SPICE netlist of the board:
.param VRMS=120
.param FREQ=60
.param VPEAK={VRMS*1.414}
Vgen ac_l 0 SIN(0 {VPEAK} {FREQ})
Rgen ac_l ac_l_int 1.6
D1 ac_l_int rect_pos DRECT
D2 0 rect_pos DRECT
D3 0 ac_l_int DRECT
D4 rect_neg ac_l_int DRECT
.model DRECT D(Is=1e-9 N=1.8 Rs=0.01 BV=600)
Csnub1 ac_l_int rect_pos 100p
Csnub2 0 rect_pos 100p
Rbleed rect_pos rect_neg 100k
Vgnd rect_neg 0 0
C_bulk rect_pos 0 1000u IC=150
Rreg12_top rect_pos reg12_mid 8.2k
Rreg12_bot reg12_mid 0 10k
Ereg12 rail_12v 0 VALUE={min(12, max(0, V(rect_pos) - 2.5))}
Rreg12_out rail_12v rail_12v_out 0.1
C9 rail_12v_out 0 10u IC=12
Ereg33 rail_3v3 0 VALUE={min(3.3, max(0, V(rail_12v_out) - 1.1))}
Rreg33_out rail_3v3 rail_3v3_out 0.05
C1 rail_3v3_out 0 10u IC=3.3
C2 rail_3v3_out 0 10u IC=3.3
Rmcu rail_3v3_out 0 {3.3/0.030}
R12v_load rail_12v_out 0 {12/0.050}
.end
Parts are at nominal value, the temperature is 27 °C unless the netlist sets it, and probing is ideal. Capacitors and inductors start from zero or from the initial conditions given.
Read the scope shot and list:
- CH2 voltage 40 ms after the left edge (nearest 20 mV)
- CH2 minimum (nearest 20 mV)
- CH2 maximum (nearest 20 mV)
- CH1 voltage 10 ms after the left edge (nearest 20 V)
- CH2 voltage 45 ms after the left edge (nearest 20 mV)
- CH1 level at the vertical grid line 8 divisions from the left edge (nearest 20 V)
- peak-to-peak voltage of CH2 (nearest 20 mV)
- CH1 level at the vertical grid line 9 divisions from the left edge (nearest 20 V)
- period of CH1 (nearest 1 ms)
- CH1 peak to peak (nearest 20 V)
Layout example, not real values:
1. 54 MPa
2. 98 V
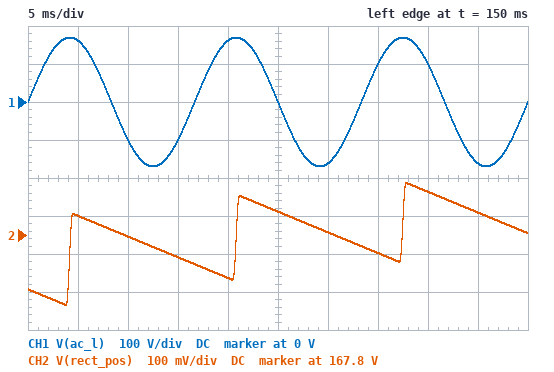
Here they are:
1. 167.92 V
2. 167.62 V
3. 167.94 V
4. -100 V
5. 167.86 V
6. 100 V
7. 320 mV
8. -160 V
9. 17 ms
10. 340 V
